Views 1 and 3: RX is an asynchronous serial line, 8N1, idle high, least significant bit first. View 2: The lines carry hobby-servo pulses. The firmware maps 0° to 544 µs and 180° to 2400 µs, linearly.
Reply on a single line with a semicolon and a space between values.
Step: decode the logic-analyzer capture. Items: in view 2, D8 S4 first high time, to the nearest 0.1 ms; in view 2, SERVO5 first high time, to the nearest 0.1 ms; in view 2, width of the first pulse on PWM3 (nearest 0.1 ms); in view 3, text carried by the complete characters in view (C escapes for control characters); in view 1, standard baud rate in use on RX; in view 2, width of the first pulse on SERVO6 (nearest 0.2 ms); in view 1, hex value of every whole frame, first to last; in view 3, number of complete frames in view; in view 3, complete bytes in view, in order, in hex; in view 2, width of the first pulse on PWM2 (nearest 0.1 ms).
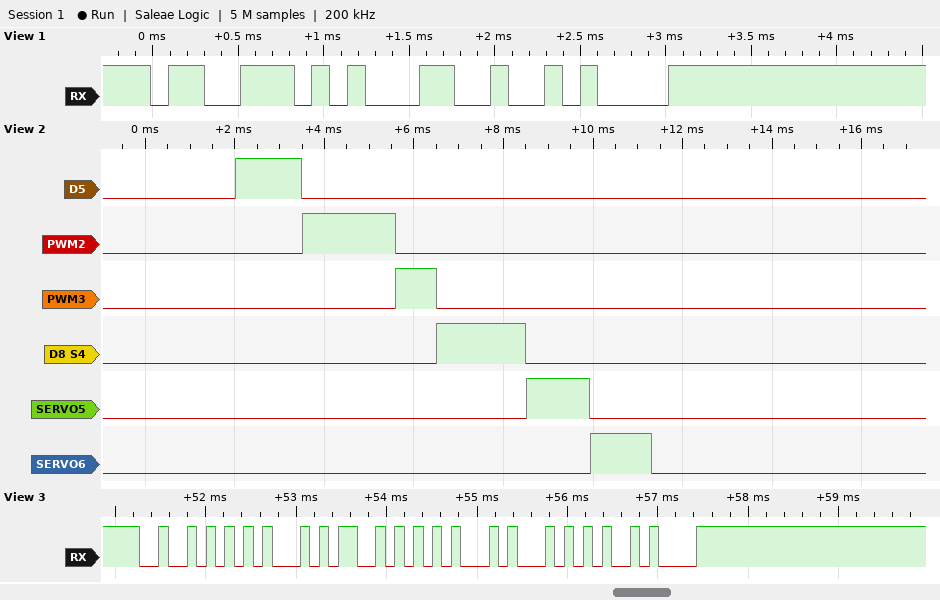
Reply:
2.0 ms; 1.4 ms; 0.9 ms; "RESET\n"; 9600 baud; 1.4 ms; 73 31 0A; 6; 52 45 53 45 54 0A; 2.1 ms
